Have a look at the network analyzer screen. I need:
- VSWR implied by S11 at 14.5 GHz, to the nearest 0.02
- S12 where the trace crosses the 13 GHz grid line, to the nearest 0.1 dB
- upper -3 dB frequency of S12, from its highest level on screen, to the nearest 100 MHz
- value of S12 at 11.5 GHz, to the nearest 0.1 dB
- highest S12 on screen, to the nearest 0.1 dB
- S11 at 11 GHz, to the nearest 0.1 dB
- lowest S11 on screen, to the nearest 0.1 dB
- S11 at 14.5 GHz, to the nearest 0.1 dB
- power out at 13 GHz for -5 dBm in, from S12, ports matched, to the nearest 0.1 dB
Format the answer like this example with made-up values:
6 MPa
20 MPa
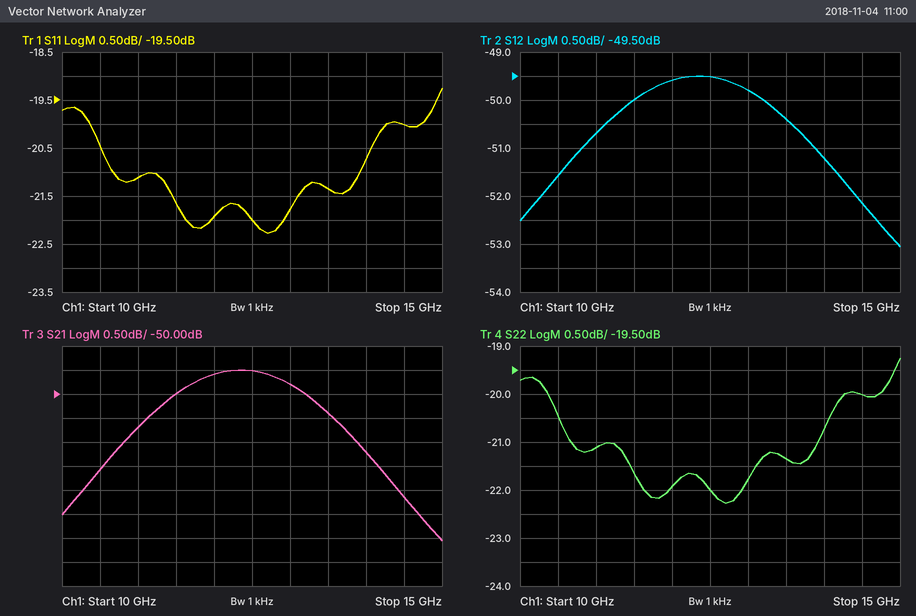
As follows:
1.22
-49.8 dB
14.7 GHz
-50.0 dB
-49.5 dB
-21.1 dB
-22.3 dB
-20.0 dB
-54.8 dBm
